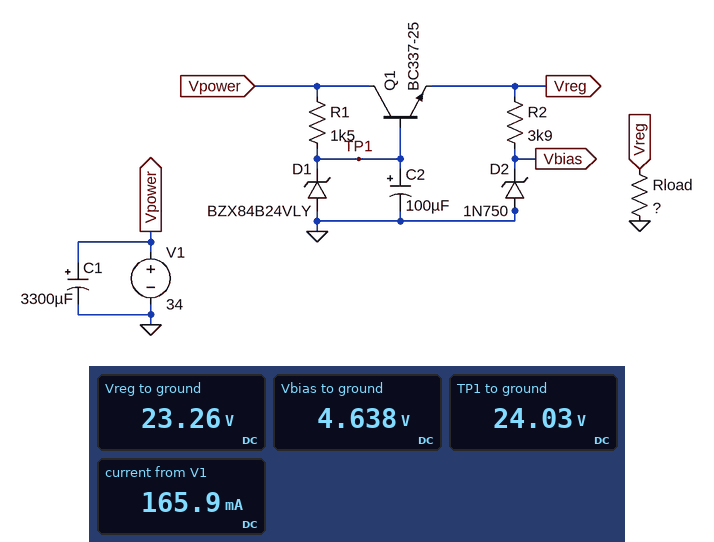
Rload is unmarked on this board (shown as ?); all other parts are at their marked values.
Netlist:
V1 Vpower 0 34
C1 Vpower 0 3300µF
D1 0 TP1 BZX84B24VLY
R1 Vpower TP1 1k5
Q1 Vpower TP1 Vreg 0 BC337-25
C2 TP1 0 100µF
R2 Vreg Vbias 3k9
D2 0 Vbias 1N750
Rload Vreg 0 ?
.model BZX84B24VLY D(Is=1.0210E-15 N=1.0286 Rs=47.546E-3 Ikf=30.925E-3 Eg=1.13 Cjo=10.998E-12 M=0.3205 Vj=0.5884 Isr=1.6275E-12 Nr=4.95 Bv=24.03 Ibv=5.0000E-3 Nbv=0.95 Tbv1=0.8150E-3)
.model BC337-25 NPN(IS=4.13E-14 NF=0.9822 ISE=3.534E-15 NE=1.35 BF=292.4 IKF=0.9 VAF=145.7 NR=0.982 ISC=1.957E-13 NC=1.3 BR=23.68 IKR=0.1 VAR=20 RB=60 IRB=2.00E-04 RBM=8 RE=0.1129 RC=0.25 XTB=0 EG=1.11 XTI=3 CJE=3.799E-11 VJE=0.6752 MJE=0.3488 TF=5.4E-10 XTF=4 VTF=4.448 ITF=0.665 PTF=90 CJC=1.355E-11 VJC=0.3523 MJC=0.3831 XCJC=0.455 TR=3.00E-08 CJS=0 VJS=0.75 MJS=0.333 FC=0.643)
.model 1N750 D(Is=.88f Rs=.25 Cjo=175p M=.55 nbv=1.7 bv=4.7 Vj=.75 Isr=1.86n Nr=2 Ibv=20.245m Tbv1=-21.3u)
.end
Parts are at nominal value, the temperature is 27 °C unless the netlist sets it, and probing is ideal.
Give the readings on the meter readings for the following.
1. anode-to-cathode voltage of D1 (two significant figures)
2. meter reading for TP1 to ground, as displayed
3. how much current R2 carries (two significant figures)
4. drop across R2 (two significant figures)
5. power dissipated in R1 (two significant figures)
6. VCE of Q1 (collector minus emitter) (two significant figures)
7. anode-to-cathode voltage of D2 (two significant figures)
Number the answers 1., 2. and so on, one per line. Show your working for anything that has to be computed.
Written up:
1. 0 V - 24.03 V = -24 V
2. 24.03 V
3. (23.26 V - 4.638 V) / 3.9 kΩ = 4.8 mA
4. 23.26 V - 4.638 V = 19 V
5. (34 V - 24.03 V)^2 / 1.5 kΩ = 66 mW
6. 34 V - 23.26 V = 11 V
7. 0 V - 4.638 V = -4.6 V
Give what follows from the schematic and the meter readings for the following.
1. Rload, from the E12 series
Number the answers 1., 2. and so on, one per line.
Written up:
1. 150 Ω
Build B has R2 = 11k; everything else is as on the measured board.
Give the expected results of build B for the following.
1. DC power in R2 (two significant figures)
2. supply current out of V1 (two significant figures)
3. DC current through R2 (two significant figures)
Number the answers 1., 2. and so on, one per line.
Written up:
1. 32 mW
2. 160 mA
3. 1.7 mA
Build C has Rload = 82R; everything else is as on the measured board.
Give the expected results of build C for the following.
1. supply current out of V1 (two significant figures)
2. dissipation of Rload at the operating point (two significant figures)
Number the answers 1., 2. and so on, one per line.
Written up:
1. 290 mA
2. 6.6 W
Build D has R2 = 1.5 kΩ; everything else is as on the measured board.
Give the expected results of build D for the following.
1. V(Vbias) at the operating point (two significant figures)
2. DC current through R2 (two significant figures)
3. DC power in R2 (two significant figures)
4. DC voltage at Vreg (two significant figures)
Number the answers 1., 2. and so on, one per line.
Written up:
1. 4.7 V
2. 12 mA
3. 230 mW
4. 23 V
